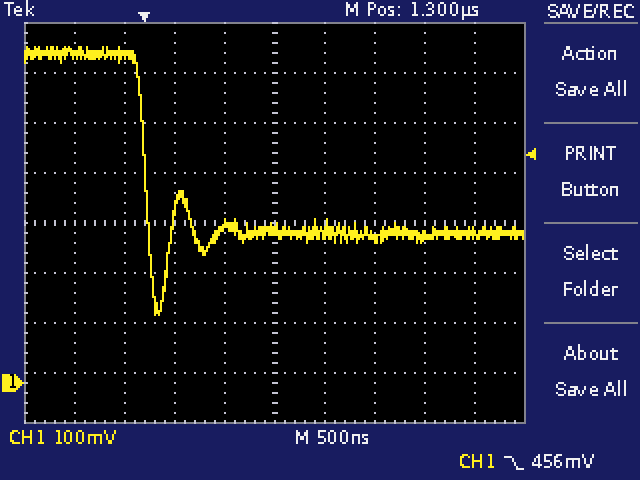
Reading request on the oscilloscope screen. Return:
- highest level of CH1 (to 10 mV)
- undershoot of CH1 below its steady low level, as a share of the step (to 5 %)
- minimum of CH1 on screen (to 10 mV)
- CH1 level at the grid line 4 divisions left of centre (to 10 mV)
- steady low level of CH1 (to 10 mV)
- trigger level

670 mV
45 %
140 mV
660 mV
300 mV
456 mV
